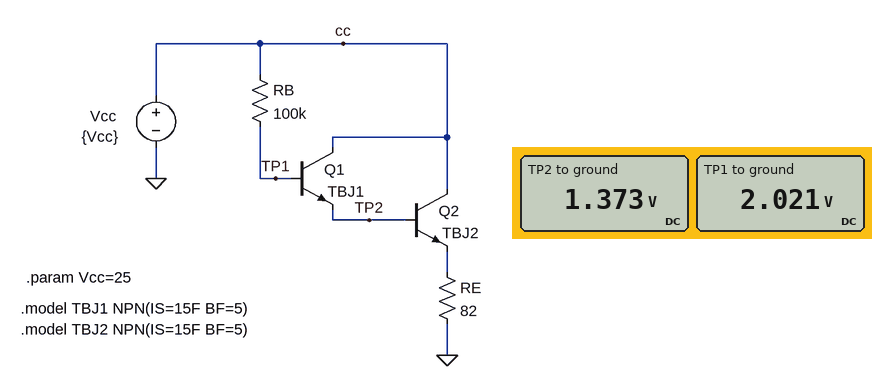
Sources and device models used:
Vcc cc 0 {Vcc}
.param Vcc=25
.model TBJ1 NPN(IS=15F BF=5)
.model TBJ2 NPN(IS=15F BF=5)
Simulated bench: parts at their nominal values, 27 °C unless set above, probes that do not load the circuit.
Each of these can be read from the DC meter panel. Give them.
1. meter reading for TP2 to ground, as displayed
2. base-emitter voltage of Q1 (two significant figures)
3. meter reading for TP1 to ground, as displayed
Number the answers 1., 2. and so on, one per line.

1. 1.373 V
2. 650 mV
3. 2.021 V
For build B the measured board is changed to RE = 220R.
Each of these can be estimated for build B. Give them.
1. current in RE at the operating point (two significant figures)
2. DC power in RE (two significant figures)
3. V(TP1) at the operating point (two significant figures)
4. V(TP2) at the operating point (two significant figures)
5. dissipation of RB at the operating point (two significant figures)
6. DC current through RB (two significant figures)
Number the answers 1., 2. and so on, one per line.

1. 7.9 mA
2. 14 mW
3. 3.1 V
4. 2.4 V
5. 4.8 mW
6. 220 µA
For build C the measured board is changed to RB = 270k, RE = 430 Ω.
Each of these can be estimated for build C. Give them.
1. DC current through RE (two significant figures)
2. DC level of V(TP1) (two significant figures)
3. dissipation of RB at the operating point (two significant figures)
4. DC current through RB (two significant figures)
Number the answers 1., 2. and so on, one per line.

1. 3.0 mA
2. 2.6 V
3. 1.9 mW
4. 83 µA
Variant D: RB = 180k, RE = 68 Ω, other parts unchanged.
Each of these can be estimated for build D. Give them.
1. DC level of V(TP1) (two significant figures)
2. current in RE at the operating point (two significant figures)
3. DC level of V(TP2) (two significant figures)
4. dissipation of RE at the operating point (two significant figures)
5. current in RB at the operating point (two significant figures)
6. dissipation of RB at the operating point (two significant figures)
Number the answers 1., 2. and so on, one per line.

1. 1.6 V
2. 4.7 mA
3. 1.0 V
4. 1.5 mW
5. 130 µA
6. 3.0 mW
